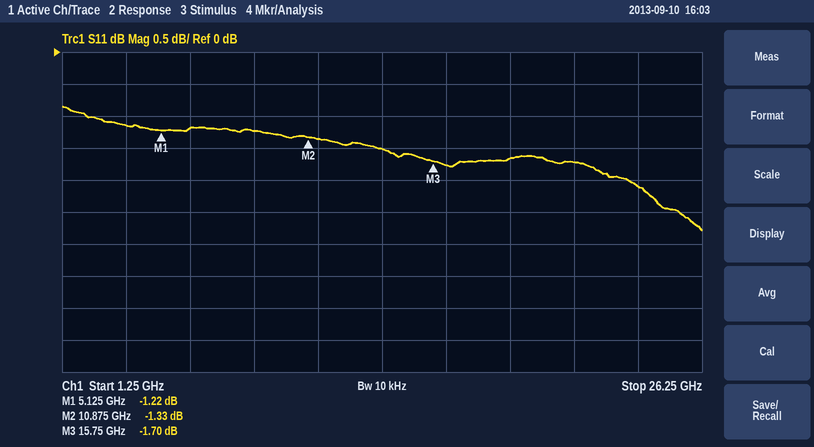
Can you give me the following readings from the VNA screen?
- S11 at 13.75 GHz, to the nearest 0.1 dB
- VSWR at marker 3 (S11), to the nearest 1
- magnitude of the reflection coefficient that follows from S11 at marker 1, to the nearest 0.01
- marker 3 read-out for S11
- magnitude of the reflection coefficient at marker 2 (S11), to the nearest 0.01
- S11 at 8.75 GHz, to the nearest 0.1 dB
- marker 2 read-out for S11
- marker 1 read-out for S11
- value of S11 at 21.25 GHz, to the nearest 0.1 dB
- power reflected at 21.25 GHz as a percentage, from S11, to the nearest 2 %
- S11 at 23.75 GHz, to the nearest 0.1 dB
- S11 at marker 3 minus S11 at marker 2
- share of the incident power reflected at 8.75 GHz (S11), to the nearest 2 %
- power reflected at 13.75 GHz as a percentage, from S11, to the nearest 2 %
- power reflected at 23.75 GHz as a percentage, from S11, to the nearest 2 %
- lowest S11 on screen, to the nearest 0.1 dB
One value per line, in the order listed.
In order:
-1.5 dB
10
0.87
-1.70 dB
0.86
-1.2 dB
-1.33 dB
-1.22 dB
-1.7 dB
68 %
-2.1 dB
-0.37 dB
76 %
70 %
62 %
-2.8 dB
